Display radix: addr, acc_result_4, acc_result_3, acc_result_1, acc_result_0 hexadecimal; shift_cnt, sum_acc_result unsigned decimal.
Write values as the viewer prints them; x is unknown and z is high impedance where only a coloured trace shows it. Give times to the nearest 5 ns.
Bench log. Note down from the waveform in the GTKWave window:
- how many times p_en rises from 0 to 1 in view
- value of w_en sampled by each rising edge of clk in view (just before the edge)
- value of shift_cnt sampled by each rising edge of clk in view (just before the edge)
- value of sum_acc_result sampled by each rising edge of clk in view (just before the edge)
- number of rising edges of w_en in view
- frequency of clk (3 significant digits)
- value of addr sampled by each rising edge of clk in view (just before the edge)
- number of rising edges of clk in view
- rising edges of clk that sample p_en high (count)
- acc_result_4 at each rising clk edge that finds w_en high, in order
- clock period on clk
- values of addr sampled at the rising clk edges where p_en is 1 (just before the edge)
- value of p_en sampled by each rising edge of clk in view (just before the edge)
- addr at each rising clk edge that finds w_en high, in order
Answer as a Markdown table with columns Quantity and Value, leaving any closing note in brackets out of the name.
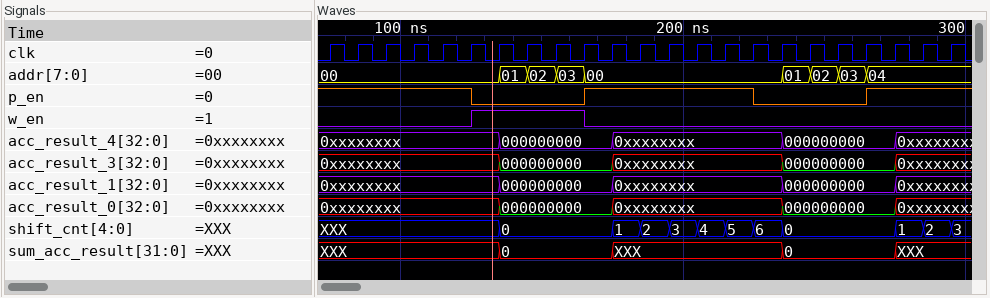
| Quantity | Value |
|---|---|
| how many times p_en rises from 0 to 1 in view | 2 |
| value of w_en sampled by each rising edge of clk in view | 0 0 0 0 0 0 1 1 1 1 0 0 0 0 0 0 0 0 0 0 0 0 0 |
| value of shift_cnt sampled by each rising edge of clk in view | XXX, XXX, XXX, XXX, XXX, XXX, XXX, 0, 0, 0, 0, 1, 2, 3, 4, 5, 6, 0, 0, 0, 0, 1, 2 |
| value of sum_acc_result sampled by each rising edge of clk in view | XXX, XXX, XXX, XXX, XXX, XXX, XXX, 0, 0, 0, 0, XXX, XXX, XXX, XXX, XXX, XXX, 0, 0, 0, 0, XXX, XXX |
| number of rising edges of w_en in view | 1 |
| frequency of clk | 100 MHz |
| value of addr sampled by each rising edge of clk in view | 00, 00, 00, 00, 00, 00, 00, 01, 02, 03, 00, 00, 00, 00, 00, 00, 00, 01, 02, 03, 04, 04, 04 |
| number of rising edges of clk in view | 23 |
| rising edges of clk that sample p_en high | 15 |
| acc_result_4 at each rising clk edge that finds w_en high, in order | 0xxxxxxxx, 000000000, 000000000, 000000000 |
| clock period on clk | 10 ns |
| values of addr sampled at the rising clk edges where p_en is 1 | 00, 00, 00, 00, 00, 00, 00, 00, 00, 00, 00, 00, 04, 04, 04 |
| value of p_en sampled by each rising edge of clk in view | 1 1 1 1 1 1 0 0 0 0 1 1 1 1 1 1 0 0 0 0 1 1 1 |
| addr at each rising clk edge that finds w_en high, in order | 00, 01, 02, 03 |
